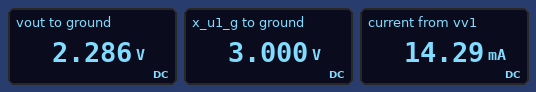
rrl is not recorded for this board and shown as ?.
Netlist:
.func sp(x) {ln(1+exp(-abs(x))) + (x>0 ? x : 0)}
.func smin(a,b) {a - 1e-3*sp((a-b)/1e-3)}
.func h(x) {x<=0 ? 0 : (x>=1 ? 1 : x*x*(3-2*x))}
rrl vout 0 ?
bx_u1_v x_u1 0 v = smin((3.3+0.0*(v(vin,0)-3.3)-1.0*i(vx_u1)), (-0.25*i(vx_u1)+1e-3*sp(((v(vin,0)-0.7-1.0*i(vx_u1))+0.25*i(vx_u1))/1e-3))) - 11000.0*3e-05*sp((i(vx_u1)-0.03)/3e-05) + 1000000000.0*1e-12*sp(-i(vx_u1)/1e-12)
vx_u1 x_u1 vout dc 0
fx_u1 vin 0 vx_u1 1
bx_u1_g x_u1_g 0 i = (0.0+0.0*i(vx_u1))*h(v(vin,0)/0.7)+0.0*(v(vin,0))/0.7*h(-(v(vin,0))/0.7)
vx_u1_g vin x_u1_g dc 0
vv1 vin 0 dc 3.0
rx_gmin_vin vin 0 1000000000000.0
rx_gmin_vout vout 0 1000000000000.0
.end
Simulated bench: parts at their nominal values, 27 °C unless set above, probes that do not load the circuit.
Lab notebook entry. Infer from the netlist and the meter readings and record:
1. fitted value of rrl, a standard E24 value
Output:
160 Ω
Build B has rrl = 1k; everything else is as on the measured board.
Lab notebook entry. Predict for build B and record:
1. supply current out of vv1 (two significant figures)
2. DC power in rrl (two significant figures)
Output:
2.3 mA
5.3 mW
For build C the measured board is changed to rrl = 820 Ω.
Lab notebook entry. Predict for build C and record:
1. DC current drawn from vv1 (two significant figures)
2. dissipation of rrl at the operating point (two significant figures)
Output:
2.8 mA
6.4 mW
